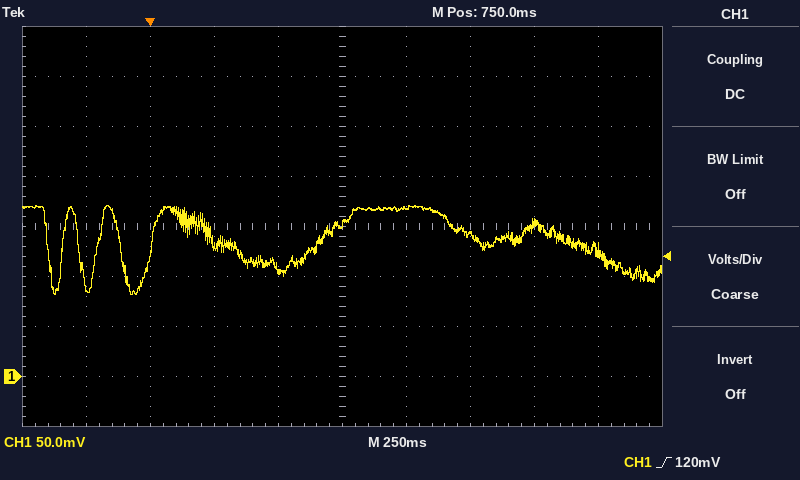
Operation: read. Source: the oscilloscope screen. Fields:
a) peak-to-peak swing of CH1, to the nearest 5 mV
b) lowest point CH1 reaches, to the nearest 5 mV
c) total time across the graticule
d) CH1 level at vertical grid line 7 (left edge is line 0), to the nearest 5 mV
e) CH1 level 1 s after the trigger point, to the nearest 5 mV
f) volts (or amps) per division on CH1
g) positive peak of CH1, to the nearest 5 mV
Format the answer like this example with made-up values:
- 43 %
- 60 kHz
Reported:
- 90 mV
- 80 mV
- 2.5 s
- 140 mV
- 170 mV
- 50 mV
- 170 mV
